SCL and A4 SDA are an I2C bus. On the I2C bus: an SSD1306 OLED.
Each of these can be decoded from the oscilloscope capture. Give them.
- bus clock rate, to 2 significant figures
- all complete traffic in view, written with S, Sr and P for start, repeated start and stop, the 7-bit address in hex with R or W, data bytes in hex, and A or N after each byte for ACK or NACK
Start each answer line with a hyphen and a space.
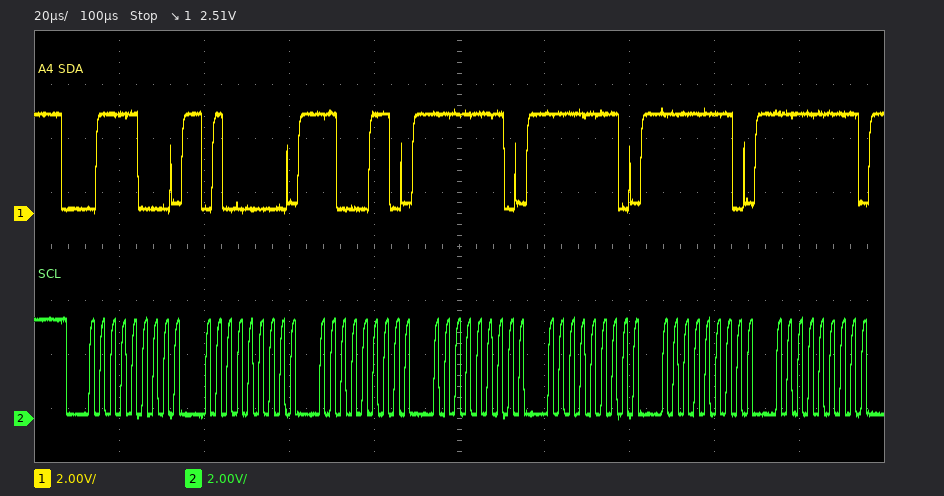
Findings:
- 400 kHz
- S 3CW A 40 A C6 A FE A FE A FE A FF A
